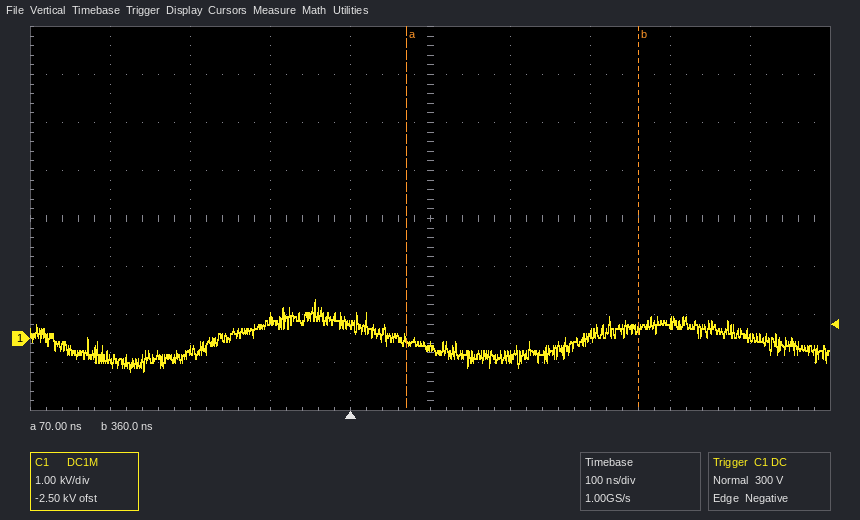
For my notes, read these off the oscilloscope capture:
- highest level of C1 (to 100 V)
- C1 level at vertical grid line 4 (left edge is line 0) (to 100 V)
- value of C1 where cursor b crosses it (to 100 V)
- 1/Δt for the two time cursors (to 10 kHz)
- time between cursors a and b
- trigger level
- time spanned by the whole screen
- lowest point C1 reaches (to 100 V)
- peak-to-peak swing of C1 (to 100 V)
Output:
800 V
300 V
200 V
3.45 MHz
290 ns
300 V
1 µs
-700 V
1.5 kV
